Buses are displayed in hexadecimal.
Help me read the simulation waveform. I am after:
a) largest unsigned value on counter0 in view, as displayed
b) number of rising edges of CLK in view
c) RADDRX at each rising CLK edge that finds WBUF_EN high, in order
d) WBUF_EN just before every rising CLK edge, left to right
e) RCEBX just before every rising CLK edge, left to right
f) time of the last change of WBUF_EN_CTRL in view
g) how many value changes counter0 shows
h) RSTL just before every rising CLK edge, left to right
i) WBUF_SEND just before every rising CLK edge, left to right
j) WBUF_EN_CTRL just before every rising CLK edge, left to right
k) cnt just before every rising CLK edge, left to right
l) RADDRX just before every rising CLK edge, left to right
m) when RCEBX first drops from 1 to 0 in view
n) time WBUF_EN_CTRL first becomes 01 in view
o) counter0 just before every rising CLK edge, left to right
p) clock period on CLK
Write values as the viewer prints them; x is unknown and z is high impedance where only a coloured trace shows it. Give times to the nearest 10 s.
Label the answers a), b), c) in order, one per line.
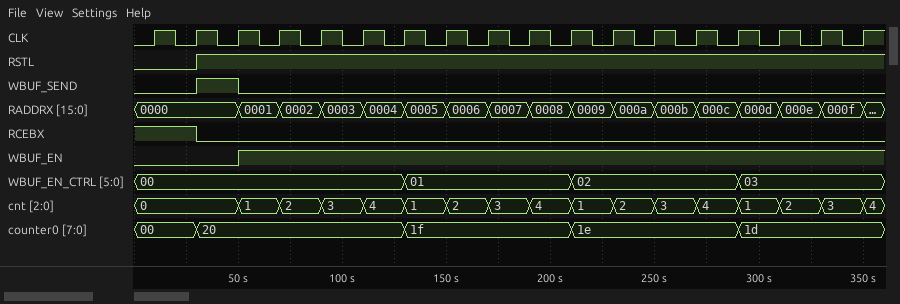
a) 20
b) 18
c) 0001, 0002, 0003, 0004, 0005, 0006, 0007, 0008, 0009, 000a, 000b, 000c, 000d, 000e, 000f
d) 0 0 0 1 1 1 1 1 1 1 1 1 1 1 1 1 1 1
e) 1 1 0 0 0 0 0 0 0 0 0 0 0 0 0 0 0 0
f) 290 s
g) 4
h) 0 0 1 1 1 1 1 1 1 1 1 1 1 1 1 1 1 1
i) 0 0 1 0 0 0 0 0 0 0 0 0 0 0 0 0 0 0
j) 00, 00, 00, 00, 00, 00, 00, 01, 01, 01, 01, 02, 02, 02, 02, 03, 03, 03
k) 0, 0, 0, 1, 2, 3, 4, 1, 2, 3, 4, 1, 2, 3, 4, 1, 2, 3
l) 0000, 0000, 0000, 0001, 0002, 0003, 0004, 0005, 0006, 0007, 0008, 0009, 000a, 000b, 000c, 000d, 000e, 000f
m) 30 s
n) 130 s
o) 00, 00, 20, 20, 20, 20, 20, 1f, 1f, 1f, 1f, 1e, 1e, 1e, 1e, 1d, 1d, 1d
p) 20 s
